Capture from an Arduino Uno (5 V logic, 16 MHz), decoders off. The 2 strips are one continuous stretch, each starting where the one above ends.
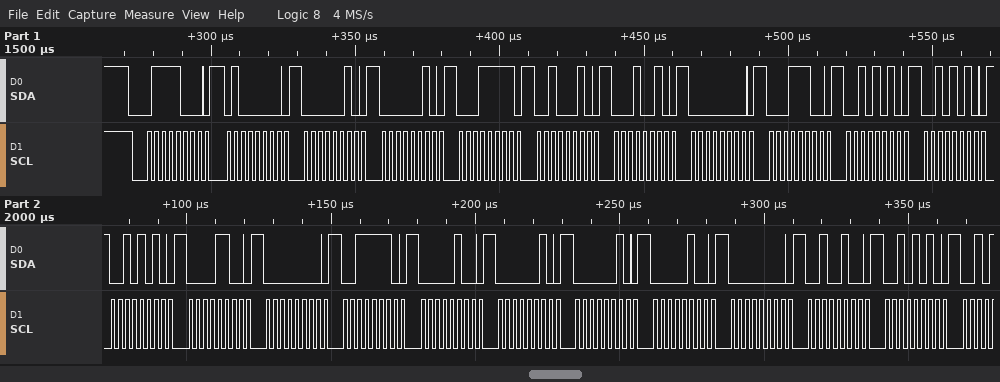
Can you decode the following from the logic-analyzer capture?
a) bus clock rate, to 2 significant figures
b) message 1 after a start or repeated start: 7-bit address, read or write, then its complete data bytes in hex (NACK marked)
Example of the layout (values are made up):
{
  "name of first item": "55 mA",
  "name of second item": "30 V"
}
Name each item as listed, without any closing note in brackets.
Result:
{
  "bus clock rate, to 2 significant figures": "400 kHz",
  "message 1 after a start or repeated start: 7-bit address, read or write, then its complete data bytes in hex": "0x3C write: 40 02 02 1F 22 12 00 1C 2A 2A 2A 0C 00 3E 04 02 02 04 00 24 2A"
}
